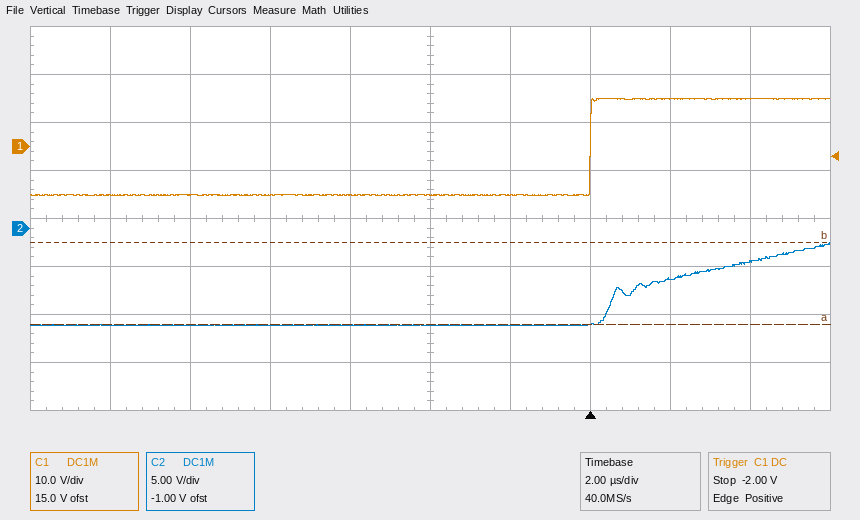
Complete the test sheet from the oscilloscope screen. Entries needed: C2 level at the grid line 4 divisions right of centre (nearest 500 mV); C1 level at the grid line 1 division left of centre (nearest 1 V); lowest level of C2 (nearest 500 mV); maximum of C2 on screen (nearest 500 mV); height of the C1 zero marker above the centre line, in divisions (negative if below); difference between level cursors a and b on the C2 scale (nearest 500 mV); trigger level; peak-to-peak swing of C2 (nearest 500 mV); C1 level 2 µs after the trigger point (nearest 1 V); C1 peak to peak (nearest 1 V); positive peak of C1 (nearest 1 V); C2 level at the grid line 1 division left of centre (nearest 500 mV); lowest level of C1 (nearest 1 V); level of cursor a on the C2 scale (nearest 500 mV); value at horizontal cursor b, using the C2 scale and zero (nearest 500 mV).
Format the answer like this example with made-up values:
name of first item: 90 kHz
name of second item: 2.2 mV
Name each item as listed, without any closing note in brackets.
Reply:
C2 level at the grid line 4 divisions right of centre: -3.5 V
C1 level at the grid line 1 division left of centre: -10 V
lowest level of C2: -10.0 V
maximum of C2 on screen: -1.5 V
height of the C1 zero marker above the centre line, in divisions: +1.5 div
difference between level cursors a and b on the C2 scale: 8.5 V
trigger level: -2.00 V
peak-to-peak swing of C2: 8.5 V
C1 level 2 µs after the trigger point: 10 V
C1 peak to peak: 20 V
positive peak of C1: 10 V
C2 level at the grid line 1 division left of centre: -10.0 V
lowest level of C1: -10 V
level of cursor a on the C2 scale: -10.0 V
value at horizontal cursor b, using the C2 scale and zero: -1.5 V
